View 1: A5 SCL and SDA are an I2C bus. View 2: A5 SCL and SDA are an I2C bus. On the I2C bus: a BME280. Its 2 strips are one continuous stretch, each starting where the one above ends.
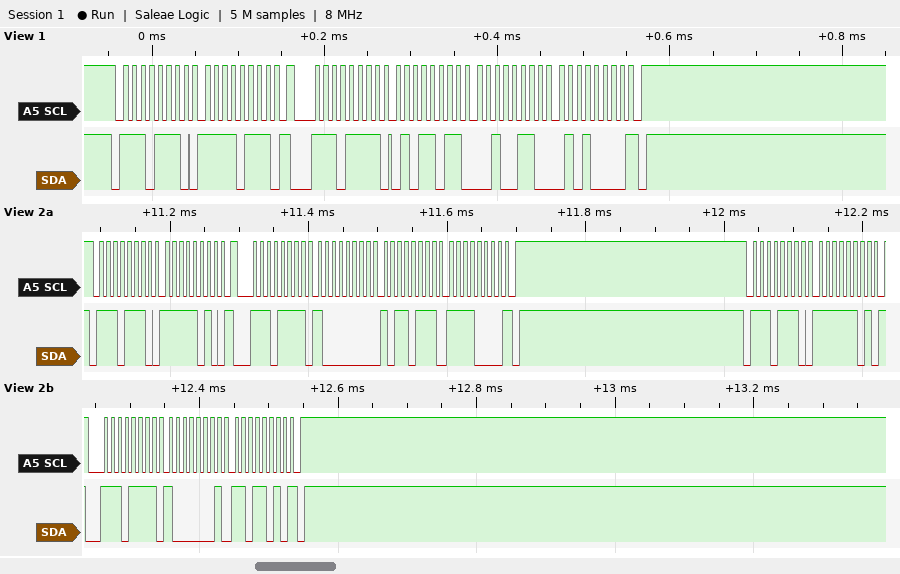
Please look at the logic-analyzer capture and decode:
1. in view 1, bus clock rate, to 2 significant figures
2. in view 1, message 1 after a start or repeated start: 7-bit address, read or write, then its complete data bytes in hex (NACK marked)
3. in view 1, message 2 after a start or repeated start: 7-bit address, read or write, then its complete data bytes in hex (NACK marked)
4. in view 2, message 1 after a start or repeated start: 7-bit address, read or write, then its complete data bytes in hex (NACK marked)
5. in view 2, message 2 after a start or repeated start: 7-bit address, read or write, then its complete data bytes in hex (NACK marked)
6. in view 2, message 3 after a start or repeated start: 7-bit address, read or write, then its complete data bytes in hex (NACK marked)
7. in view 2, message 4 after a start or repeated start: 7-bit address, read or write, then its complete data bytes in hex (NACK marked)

100 kHz
0x77 write: F7
0x77 read: 5B 26 50 NACK
0x77 write: FA
0x77 read: 80 B7 F0 NACK
0x77 write: FD
0x77 read: 81 DA NACK
